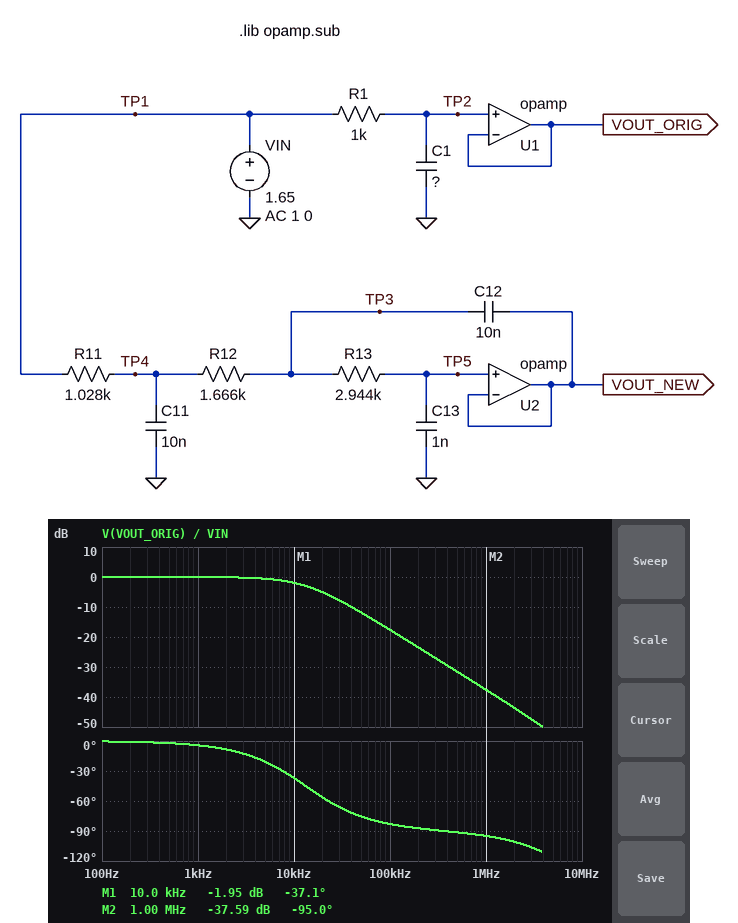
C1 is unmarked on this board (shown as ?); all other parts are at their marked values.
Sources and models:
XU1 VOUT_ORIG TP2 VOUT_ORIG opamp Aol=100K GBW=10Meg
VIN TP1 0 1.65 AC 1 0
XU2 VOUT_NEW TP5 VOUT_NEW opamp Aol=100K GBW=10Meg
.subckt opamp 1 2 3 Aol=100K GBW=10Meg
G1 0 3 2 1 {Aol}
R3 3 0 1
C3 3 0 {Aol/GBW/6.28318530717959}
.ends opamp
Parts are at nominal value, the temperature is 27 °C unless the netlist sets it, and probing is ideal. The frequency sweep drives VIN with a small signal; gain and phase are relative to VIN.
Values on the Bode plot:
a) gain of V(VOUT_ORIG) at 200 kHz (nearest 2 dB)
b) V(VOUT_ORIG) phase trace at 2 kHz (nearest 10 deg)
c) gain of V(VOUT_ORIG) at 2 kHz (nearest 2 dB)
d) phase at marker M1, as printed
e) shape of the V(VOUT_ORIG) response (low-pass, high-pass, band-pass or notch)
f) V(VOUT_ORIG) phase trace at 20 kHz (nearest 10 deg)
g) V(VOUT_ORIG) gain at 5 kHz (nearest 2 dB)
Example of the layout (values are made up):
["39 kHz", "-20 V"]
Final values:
["-24 dB", "-10 deg", "0 dB", "-37.1 deg", "low-pass", "-60 deg", "0 dB"]
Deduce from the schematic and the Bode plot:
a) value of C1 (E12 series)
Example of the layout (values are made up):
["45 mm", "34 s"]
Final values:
["12 nF"]
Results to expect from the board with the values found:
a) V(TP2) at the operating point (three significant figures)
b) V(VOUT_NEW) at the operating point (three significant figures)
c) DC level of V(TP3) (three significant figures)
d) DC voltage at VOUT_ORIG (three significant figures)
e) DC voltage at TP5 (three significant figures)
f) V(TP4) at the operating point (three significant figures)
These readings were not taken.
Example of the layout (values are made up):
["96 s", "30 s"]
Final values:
["1.65 V", "1.65 V", "1.65 V", "1.65 V", "1.65 V", "1.65 V"]
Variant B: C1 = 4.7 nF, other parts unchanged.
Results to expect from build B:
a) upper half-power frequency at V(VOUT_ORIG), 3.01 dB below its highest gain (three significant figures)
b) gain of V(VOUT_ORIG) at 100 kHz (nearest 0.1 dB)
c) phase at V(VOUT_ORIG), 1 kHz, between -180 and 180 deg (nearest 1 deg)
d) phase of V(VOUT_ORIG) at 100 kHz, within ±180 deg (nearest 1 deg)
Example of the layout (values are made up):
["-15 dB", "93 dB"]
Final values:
["33.9 kHz", "-9.9 dB", "-2 deg", "-72 deg"]
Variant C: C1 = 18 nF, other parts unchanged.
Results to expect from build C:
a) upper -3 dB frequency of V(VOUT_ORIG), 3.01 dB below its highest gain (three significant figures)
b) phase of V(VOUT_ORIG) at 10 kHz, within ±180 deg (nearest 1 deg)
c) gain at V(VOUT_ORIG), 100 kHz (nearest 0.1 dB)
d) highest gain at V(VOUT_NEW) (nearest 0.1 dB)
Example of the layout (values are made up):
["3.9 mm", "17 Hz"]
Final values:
["8.84 kHz", "-49 deg", "-21.1 dB", "0 dB"]
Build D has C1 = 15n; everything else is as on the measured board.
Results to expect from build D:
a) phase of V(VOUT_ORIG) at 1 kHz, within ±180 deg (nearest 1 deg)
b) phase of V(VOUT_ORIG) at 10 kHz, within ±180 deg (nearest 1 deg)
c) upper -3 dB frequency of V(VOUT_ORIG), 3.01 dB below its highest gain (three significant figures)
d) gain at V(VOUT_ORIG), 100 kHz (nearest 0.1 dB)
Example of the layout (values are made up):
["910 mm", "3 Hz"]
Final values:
["-5 deg", "-43 deg", "10.6 kHz", "-19.5 dB"]
